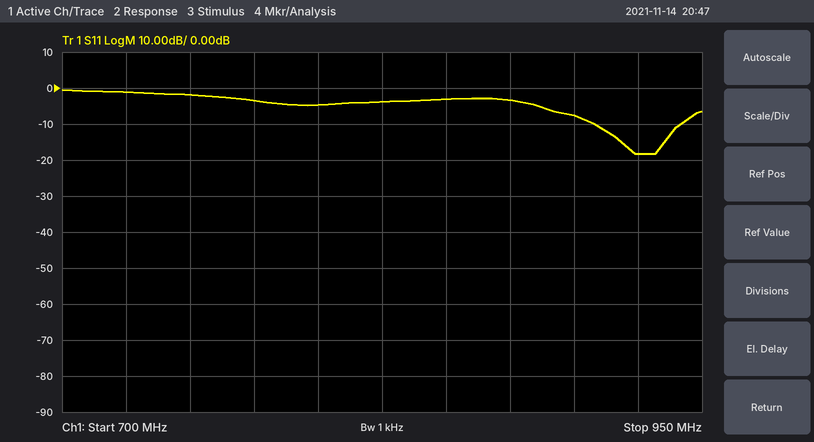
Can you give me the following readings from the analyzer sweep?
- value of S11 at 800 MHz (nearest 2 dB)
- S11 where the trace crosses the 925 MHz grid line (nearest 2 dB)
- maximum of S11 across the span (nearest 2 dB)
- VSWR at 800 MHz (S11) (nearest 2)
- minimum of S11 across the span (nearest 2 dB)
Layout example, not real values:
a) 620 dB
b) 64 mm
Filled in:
a) -4 dB
b) -18 dB
c) 0 dB
d) 4
e) -18 dB
